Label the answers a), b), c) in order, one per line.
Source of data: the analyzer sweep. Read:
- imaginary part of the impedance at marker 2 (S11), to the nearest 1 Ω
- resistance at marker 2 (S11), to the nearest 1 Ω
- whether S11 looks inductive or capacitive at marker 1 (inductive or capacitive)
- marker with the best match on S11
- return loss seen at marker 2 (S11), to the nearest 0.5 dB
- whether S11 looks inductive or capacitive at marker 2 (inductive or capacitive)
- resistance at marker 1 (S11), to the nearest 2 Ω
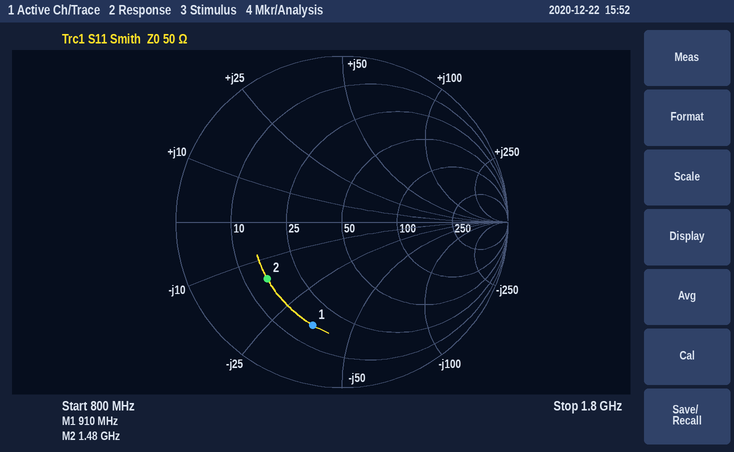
a) -15 Ω
b) 15 Ω
c) capacitive
d) marker 2
e) 5.0 dB
f) capacitive
g) 16 Ω
